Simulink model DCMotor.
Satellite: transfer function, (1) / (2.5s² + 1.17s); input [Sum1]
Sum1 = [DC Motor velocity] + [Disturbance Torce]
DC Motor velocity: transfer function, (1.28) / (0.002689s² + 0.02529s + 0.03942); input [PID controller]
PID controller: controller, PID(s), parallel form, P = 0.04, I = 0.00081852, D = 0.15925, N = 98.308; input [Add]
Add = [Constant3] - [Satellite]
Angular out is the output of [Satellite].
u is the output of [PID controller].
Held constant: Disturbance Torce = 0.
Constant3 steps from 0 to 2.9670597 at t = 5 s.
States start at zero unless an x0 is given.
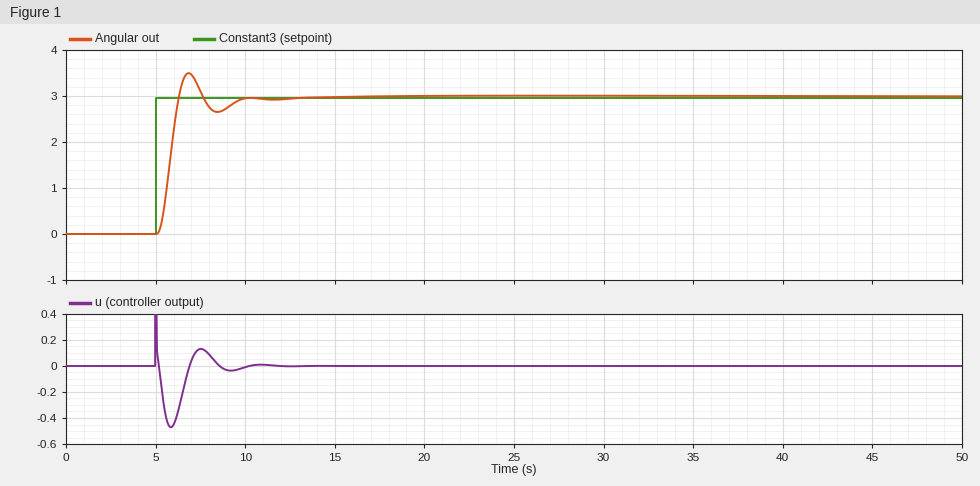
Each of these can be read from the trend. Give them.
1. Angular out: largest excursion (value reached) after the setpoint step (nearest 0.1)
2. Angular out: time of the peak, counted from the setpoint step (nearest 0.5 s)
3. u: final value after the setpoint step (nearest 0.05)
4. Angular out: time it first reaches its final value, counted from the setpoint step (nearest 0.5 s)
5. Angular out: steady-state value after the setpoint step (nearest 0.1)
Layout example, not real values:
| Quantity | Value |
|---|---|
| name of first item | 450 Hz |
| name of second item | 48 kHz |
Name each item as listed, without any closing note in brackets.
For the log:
| Quantity | Value |
|---|---|
| Angular out: largest excursion (value reached) after the setpoint step | 3.5 |
| Angular out: time of the peak, counted from the setpoint step | 2.0 s |
| u: final value after the setpoint step | 0.00 |
| Angular out: time it first reaches its final value, counted from the setpoint step | 1.5 s |
| Angular out: steady-state value after the setpoint step | 3.0 |
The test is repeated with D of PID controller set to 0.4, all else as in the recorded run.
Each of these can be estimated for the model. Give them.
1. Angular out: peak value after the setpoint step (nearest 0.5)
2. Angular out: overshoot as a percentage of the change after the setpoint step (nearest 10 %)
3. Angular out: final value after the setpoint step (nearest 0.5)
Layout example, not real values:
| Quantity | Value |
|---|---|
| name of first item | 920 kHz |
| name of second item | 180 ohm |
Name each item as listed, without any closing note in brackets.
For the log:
| Quantity | Value |
|---|---|
| Angular out: peak value after the setpoint step | 4.5 |
| Angular out: overshoot as a percentage of the change after the setpoint step | 50 % |
| Angular out: final value after the setpoint step | 3.0 |
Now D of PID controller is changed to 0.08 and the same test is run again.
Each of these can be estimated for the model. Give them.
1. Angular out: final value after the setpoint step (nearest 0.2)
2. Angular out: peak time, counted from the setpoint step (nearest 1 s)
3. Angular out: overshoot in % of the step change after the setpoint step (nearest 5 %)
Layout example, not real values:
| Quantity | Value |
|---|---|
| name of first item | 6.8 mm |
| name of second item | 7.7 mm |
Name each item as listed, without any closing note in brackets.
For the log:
| Quantity | Value |
|---|---|
| Angular out: final value after the setpoint step | 3.0 |
| Angular out: peak time, counted from the setpoint step | 3 s |
| Angular out: overshoot in % of the step change after the setpoint step | 15 % |
